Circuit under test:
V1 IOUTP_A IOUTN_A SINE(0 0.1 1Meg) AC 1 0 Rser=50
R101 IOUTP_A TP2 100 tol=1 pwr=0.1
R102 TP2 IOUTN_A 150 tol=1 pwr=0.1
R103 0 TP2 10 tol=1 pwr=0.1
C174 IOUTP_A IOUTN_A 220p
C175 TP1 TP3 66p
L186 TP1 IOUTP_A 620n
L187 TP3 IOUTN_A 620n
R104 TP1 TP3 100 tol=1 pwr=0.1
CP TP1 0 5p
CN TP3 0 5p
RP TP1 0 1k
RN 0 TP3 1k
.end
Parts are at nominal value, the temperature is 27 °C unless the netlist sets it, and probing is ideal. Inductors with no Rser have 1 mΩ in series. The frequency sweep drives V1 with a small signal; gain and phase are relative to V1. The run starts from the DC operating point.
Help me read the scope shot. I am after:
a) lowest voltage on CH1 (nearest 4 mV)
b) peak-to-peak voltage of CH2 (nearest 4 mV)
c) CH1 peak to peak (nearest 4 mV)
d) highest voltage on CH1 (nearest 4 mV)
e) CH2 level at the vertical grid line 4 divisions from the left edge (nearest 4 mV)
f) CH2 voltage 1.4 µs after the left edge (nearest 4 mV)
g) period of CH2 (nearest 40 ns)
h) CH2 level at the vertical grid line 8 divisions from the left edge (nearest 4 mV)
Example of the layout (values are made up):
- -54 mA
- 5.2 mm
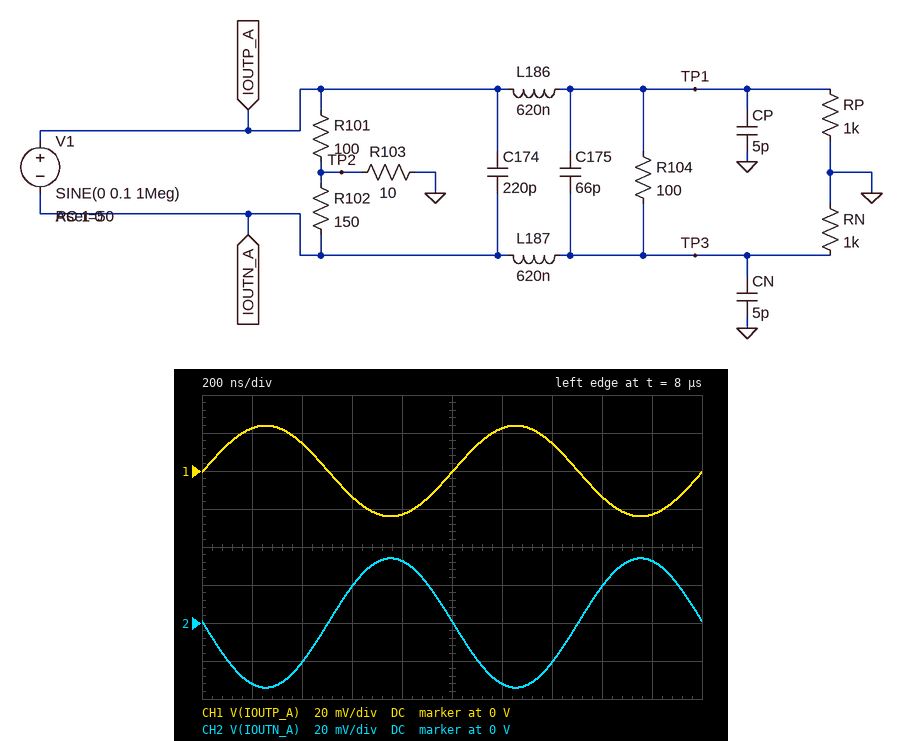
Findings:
- -24 mV
- 68 mV
- 48 mV
- 24 mV
- 32 mV
- -20 mV
- 1.00 µs
- 20 mV
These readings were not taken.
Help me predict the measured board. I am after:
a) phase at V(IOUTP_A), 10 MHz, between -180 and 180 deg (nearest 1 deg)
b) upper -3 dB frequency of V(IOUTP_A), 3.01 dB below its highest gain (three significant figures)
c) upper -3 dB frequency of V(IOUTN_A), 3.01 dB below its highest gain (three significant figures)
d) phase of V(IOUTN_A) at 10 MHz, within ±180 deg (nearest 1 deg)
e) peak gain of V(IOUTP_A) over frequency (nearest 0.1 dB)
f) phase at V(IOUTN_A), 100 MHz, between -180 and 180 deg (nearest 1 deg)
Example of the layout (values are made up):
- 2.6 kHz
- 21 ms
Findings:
- -14 deg
- 32.9 MHz
- 32.4 MHz
- 165 deg
- -12.2 dB
- 102 deg
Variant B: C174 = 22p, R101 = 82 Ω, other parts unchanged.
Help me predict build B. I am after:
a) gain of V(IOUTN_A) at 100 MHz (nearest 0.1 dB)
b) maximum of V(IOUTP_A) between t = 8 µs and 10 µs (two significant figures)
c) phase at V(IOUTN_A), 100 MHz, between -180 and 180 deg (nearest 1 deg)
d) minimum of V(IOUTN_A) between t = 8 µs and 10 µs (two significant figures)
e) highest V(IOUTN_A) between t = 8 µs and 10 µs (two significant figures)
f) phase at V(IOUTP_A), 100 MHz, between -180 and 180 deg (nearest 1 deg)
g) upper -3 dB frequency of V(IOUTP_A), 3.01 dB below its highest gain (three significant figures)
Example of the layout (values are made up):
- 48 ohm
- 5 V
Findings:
- -7.5 dB
- 21 mV
- 156 deg
- -36 mV
- 36 mV
- -31 deg
- 161 MHz
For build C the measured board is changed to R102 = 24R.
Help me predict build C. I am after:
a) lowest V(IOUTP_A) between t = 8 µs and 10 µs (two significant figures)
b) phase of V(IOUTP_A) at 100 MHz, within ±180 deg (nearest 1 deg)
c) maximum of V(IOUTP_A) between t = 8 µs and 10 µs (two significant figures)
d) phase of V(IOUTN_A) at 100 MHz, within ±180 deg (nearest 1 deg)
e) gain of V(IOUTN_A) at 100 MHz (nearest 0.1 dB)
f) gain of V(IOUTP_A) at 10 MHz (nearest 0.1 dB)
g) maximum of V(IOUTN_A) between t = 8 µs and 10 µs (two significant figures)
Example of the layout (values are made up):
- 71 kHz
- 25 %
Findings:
- -41 mV
- -74 deg
- 41 mV
- 91 deg
- -27.9 dB
- -7.8 dB
- 11 mV
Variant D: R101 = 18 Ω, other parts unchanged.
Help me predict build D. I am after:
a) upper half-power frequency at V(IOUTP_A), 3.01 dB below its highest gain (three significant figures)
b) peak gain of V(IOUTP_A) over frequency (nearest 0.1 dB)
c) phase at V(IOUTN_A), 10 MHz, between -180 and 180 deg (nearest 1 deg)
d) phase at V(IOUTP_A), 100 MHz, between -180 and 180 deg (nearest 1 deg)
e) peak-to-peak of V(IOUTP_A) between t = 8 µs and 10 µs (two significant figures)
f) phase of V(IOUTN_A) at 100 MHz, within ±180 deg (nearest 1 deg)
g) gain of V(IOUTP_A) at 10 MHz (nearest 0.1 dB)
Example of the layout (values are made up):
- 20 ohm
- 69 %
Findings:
- 36.1 MHz
- -22.8 dB
- 166 deg
- -97 deg
- 14 mV
- 106 deg
- -23.2 dB
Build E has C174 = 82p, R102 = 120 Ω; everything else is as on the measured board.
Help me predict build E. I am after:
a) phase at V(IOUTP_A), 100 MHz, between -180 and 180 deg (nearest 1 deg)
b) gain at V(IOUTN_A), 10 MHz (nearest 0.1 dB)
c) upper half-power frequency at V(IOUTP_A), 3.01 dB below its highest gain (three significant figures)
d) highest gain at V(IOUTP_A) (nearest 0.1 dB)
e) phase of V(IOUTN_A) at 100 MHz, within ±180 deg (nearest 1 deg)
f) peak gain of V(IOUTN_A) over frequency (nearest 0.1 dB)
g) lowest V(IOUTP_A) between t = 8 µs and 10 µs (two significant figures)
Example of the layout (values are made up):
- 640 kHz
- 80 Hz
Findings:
- -65 deg
- -10.0 dB
- 63.7 MHz
- -9.4 dB
- 117 deg
- -8.1 dB
- -26 mV
